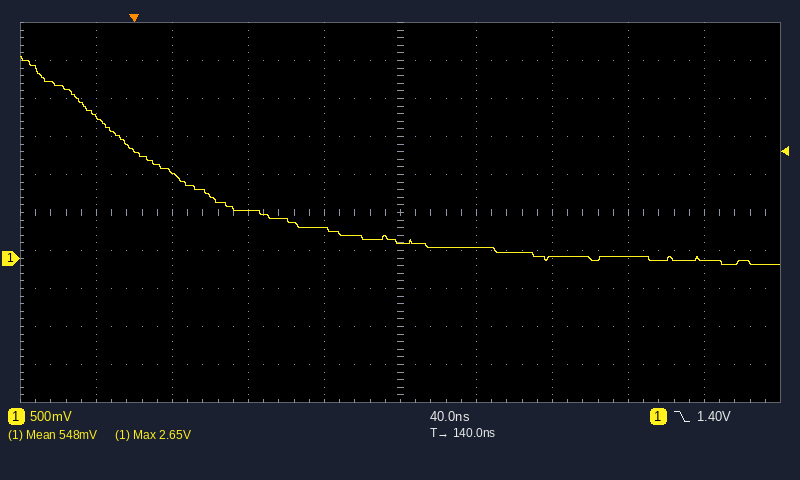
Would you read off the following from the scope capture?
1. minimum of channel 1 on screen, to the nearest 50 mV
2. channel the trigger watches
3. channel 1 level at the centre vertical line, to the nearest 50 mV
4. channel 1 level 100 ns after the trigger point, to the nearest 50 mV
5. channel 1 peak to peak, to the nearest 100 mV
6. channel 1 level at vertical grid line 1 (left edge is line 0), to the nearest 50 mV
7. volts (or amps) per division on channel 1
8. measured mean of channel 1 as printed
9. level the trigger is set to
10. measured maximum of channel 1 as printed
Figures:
-100 mV
channel 1
200 mV
400 mV
2.70 V
1.85 V
500 mV
548 mV
1.40 V
2.65 V
